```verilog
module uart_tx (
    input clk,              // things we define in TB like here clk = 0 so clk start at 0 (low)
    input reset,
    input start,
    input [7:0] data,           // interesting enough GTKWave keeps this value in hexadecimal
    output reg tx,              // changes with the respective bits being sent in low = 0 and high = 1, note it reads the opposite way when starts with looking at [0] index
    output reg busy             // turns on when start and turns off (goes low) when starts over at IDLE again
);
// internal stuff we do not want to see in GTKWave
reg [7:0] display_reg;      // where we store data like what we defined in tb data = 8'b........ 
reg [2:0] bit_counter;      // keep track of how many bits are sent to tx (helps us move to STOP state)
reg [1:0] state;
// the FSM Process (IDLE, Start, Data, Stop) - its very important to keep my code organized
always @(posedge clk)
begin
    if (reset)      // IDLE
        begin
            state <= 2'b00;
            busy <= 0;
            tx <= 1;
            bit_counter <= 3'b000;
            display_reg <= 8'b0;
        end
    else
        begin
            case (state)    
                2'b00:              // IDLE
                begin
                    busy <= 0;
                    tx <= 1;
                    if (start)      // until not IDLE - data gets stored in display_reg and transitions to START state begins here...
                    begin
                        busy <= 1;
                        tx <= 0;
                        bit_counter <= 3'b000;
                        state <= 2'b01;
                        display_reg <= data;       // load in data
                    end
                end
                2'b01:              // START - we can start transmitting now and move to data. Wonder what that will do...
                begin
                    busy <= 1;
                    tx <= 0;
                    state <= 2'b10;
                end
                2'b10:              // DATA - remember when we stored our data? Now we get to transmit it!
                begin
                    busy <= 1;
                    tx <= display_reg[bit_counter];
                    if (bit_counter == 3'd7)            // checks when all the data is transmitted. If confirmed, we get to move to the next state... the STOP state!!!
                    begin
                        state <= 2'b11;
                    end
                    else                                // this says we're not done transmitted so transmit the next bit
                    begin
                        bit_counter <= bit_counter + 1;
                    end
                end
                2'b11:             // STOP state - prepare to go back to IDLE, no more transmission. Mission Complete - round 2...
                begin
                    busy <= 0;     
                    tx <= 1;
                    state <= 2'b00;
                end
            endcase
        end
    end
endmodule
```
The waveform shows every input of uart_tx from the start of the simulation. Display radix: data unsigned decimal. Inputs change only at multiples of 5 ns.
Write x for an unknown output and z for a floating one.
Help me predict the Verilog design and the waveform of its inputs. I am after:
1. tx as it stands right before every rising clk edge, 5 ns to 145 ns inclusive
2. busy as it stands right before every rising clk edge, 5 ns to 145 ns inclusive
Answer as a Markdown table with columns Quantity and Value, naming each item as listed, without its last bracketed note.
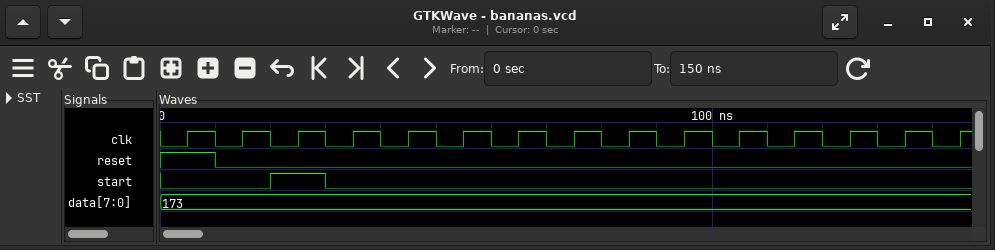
| Quantity | Value |
|---|---|
| tx as it stands right before every rising clk edge, 5 ns to 145 ns inclusive | x 1 1 0 0 1 0 1 1 0 1 0 1 1 1 |
| busy as it stands right before every rising clk edge, 5 ns to 145 ns inclusive | x 0 0 1 1 1 1 1 1 1 1 1 1 0 0 |
